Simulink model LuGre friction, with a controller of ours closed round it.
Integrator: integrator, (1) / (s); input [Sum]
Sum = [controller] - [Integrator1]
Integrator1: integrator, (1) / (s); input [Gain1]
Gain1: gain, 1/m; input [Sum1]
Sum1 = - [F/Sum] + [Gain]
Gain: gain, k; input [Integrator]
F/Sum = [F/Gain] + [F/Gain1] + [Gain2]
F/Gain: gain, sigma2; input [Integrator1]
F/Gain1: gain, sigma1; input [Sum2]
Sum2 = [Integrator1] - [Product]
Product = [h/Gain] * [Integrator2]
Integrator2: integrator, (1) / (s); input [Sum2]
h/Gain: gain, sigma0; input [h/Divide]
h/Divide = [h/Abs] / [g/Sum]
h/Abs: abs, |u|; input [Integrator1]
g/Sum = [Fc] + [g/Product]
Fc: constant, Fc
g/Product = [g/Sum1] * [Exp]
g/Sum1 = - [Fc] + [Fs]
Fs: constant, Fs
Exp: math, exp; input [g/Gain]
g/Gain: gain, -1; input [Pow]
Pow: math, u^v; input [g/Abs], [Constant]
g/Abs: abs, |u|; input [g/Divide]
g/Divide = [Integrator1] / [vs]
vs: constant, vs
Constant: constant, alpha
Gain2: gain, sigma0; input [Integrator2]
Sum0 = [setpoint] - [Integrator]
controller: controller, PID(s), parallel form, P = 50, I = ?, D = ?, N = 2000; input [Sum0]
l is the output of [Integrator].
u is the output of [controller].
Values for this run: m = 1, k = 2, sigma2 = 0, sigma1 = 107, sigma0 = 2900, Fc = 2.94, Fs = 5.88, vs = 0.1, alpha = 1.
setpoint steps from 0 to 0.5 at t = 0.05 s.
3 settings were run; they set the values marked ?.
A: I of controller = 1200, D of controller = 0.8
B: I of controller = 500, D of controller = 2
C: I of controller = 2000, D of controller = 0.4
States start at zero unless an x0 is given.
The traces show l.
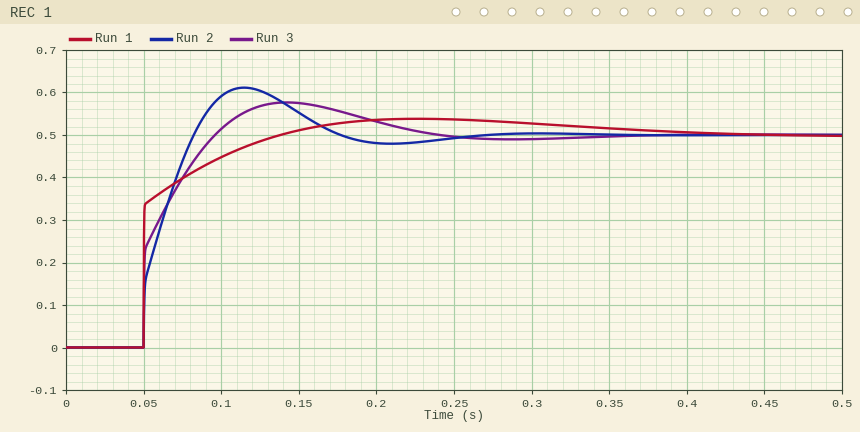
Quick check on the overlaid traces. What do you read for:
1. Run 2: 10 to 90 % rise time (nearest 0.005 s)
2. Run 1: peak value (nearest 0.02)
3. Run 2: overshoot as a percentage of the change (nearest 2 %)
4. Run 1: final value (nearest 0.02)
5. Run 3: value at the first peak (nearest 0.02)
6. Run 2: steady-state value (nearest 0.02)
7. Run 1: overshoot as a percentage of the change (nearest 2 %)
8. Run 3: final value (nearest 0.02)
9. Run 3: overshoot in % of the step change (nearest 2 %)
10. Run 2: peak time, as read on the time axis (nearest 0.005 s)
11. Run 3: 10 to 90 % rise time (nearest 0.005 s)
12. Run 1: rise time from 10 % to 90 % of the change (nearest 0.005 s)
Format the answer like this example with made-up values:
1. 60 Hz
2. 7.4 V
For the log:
1. 0.025 s
2. 0.54
3. 22 %
4. 0.50
5. 0.58
6. 0.50
7. 8 %
8. 0.50
9. 16 %
10. 0.115 s
11. 0.035 s
12. 0.050 s
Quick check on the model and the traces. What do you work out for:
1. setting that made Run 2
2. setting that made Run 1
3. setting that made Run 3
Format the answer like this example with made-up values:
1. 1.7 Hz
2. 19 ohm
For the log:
1. C
2. B
3. A
